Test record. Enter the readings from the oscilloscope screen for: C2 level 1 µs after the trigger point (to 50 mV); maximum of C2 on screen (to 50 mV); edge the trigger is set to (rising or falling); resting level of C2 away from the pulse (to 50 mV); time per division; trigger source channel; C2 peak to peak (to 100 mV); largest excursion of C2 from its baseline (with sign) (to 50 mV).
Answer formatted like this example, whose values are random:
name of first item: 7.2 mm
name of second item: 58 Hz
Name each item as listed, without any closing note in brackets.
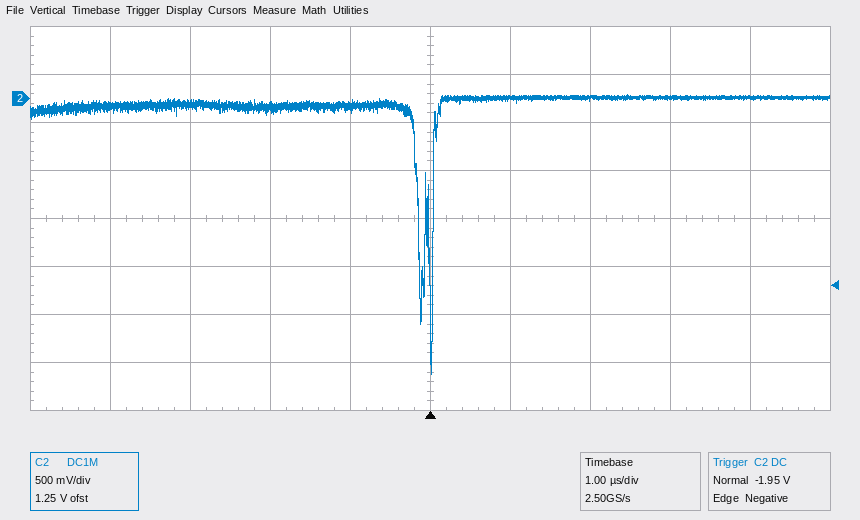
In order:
C2 level 1 µs after the trigger point: 0 mV
maximum of C2 on screen: 50 mV
edge the trigger is set to: falling
resting level of C2 away from the pulse: -50 mV
time per division: 1 µs
trigger source channel: C2
C2 peak to peak: 2.90 V
largest excursion of C2 from its baseline (with sign): -2.80 V
